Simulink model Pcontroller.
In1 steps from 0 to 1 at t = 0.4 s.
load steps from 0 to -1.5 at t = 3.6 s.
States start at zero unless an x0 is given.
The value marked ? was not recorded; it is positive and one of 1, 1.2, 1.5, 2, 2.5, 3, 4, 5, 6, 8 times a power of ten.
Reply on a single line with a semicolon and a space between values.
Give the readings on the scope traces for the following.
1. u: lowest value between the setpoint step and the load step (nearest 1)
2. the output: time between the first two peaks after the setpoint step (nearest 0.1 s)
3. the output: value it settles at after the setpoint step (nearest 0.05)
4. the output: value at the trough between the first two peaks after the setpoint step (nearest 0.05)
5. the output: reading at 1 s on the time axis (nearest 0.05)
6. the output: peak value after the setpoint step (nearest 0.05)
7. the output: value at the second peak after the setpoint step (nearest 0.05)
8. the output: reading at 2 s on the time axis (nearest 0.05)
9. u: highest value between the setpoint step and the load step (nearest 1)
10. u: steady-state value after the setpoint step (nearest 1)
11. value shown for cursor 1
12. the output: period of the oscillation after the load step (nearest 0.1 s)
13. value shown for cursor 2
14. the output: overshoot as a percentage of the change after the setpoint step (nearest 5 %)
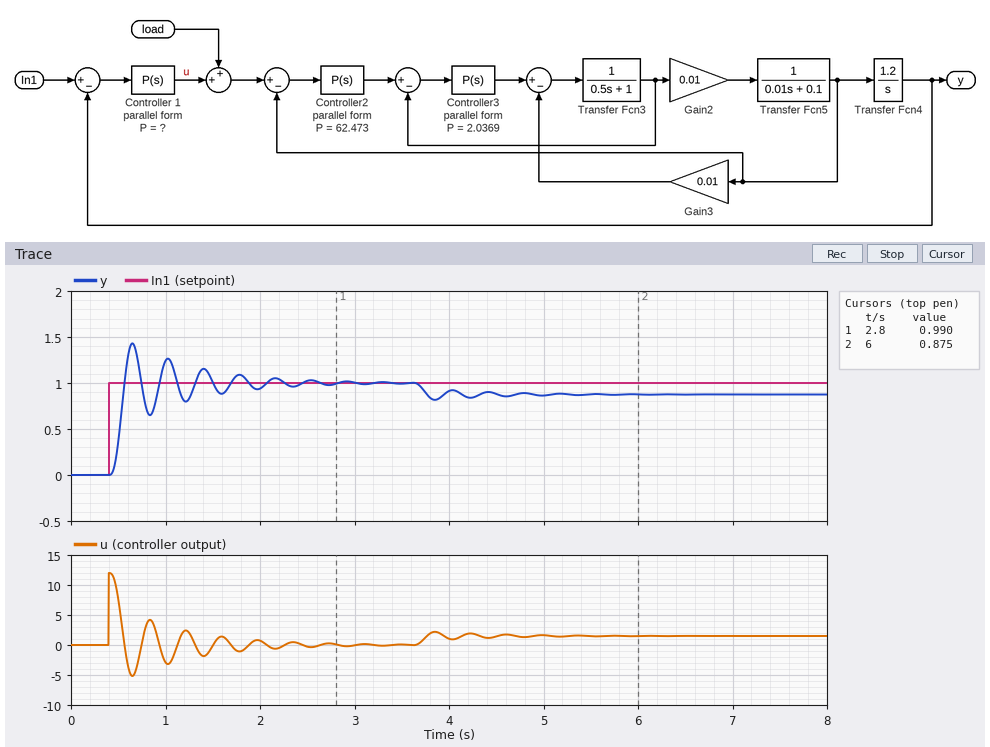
-5; 0.4 s; 1.00; 0.65; 1.25; 1.45; 1.25; 0.95; 12; 0; 0.990; 0.4 s; 0.875; 45 %
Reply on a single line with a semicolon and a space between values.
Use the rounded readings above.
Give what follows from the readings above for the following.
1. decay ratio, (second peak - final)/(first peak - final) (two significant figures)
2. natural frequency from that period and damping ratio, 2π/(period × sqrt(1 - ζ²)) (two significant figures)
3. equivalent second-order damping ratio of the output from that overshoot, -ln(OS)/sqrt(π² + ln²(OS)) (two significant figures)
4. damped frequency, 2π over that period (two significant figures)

0.56; 16 rad/s; 0.25; 16 rad/s
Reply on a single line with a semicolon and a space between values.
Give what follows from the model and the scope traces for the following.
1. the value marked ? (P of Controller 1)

12
